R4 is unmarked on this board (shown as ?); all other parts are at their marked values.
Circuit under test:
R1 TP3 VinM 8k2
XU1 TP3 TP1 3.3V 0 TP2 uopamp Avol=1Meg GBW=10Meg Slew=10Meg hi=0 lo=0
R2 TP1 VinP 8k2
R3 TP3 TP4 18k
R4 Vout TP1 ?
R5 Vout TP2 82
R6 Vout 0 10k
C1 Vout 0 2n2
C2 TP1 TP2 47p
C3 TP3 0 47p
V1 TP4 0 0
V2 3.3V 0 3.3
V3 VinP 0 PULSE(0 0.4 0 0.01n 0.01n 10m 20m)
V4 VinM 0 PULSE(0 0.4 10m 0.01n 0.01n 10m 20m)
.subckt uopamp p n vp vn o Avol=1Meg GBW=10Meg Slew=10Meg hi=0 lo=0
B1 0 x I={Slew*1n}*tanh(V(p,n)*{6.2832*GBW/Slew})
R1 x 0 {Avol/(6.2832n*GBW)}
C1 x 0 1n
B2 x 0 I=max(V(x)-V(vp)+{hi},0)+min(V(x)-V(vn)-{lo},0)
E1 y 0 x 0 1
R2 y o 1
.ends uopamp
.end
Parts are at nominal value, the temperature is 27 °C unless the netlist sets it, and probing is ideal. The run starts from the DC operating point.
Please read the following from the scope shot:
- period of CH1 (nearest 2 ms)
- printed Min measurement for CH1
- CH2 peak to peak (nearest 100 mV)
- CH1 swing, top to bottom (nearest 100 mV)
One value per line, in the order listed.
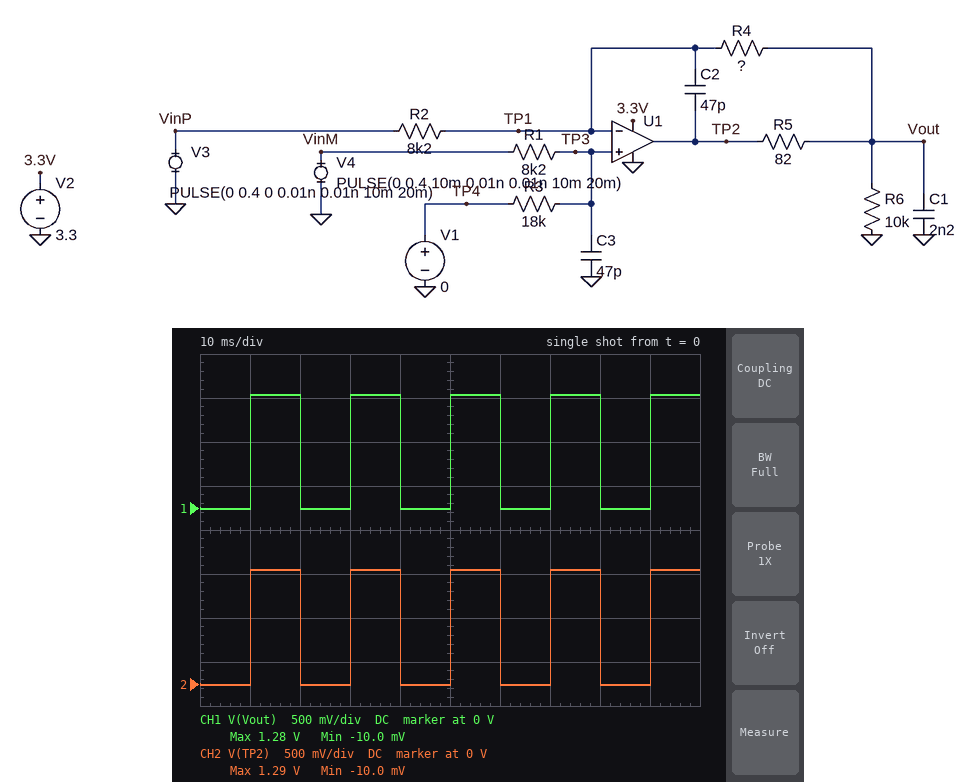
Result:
20 ms
-10.0 mV
1.3 V
1.3 V
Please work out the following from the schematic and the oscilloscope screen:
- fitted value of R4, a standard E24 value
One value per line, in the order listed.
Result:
30 kΩ
